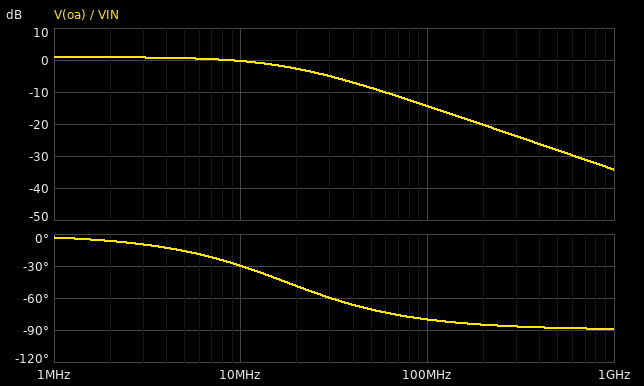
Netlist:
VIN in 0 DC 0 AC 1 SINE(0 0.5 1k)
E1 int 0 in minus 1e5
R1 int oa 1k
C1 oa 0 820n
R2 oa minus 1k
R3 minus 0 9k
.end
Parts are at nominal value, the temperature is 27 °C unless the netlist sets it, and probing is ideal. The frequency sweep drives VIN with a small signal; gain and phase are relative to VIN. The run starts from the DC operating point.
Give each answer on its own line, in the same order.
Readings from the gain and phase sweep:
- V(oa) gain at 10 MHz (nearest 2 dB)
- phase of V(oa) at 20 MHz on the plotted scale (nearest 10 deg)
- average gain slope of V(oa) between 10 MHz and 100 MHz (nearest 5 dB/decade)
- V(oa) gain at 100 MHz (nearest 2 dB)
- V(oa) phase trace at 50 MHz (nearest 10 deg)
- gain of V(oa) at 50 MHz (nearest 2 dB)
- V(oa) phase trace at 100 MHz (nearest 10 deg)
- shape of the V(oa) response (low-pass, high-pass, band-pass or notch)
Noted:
0 dB
-50 deg
-15 dB/decade
-14 dB
-70 deg
-8 dB
-80 deg
low-pass
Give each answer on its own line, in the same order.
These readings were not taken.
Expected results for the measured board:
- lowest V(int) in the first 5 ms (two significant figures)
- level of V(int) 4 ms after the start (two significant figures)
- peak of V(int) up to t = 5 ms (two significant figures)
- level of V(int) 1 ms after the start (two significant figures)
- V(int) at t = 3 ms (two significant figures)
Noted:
-2.9 V
2.9 V
2.9 V
2.9 V
2.9 V
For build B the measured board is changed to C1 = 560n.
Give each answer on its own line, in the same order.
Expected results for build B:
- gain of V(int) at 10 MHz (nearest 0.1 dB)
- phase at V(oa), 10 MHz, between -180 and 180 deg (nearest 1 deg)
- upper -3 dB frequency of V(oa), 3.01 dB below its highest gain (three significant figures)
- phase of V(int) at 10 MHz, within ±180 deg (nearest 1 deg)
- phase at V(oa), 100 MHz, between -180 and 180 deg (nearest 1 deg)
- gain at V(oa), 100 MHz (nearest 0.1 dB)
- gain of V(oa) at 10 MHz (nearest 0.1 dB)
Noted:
91.2 dB
-21 deg
25.6 MHz
69 deg
-76 deg
-11.2 dB
0.3 dB
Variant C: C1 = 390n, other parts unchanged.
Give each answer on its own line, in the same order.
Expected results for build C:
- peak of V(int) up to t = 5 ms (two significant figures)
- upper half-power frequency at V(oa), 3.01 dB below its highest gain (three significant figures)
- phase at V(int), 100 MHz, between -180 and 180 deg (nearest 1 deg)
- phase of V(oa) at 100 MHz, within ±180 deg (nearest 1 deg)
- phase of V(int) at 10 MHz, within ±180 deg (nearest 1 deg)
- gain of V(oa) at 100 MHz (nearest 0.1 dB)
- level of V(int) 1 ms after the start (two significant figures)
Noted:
1.5 V
36.7 MHz
20 deg
-70 deg
75 deg
-8.3 dB
1.4 V
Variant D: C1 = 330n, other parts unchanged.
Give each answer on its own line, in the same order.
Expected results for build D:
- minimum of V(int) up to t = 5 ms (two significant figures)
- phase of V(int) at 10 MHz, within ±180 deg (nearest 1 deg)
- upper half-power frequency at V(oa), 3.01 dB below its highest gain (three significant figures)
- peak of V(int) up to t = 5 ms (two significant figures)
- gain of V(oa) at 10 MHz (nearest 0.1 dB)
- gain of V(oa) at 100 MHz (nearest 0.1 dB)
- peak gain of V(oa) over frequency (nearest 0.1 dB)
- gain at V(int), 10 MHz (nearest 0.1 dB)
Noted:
-1.3 V
77 deg
43.4 MHz
1.3 V
0.7 dB
-7.1 dB
0.9 dB
87.0 dB
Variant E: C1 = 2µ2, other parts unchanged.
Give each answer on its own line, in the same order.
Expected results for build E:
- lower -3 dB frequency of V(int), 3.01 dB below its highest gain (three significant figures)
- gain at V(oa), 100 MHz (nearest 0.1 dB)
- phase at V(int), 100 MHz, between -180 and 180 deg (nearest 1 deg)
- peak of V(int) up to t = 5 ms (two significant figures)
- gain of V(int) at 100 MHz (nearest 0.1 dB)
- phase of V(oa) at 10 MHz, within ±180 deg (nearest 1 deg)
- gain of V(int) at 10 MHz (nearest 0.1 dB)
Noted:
6.51 MHz
-22.8 dB
4 deg
7.7 V
100.0 dB
-57 deg
98.5 dB
